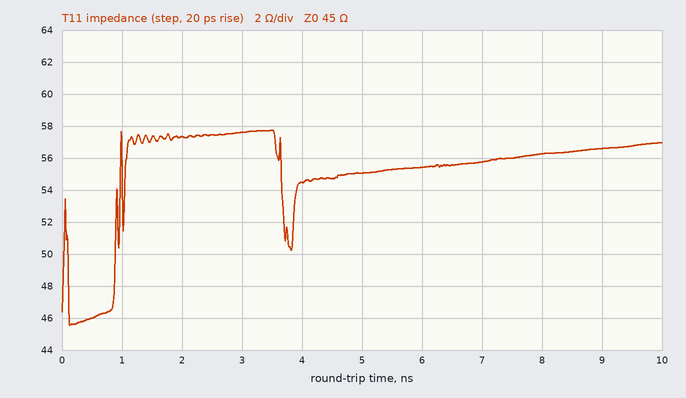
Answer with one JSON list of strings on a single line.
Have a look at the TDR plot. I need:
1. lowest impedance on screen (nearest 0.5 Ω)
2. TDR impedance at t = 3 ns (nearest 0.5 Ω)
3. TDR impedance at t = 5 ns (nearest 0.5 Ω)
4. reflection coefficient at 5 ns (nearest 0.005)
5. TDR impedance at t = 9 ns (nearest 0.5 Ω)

["45.5 Ω", "57.5 Ω", "55.0 Ω", "+0.100", "56.5 Ω"]
